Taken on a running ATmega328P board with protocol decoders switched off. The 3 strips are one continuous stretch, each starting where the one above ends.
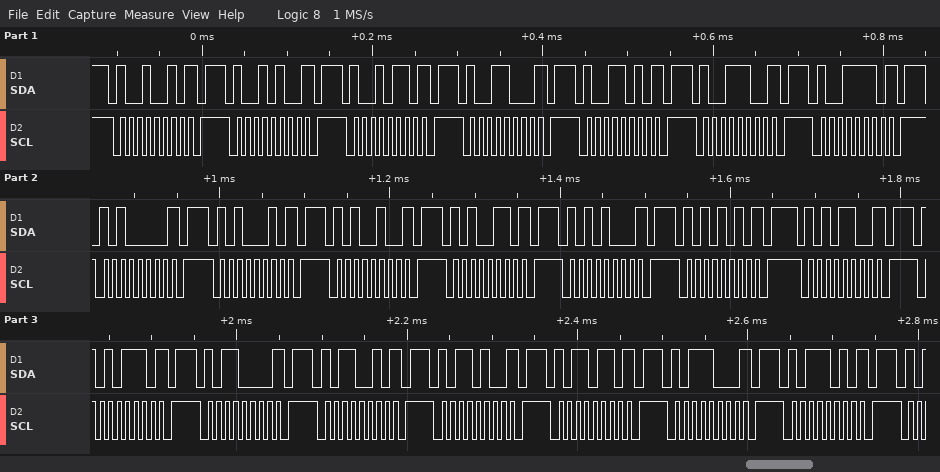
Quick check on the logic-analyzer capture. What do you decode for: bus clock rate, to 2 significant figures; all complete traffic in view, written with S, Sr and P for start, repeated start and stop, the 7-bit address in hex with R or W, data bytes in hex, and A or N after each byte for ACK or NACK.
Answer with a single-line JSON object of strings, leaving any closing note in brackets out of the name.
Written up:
{"bus clock rate, to 2 significant figures": "100 kHz", "all complete traffic in view, written with S, Sr and P for start, repeated start and stop, the 7-bit address in hex with R or W, data bytes in hex, and A or N after each byte for ACK or NACK": "S 49W N P S 4AW N P S 4BW N P S 4CW N P S 4DW N P S 4EW N P S 4FW N P S 50W N P S 51W N P S 52W N P S 53W N P S 54W N P S 55W N P S 56W N P S 57W N P S 58W N P S 59W N P S 5AW N P S 5BW N P S 5CW N P S 5DW N P"}
